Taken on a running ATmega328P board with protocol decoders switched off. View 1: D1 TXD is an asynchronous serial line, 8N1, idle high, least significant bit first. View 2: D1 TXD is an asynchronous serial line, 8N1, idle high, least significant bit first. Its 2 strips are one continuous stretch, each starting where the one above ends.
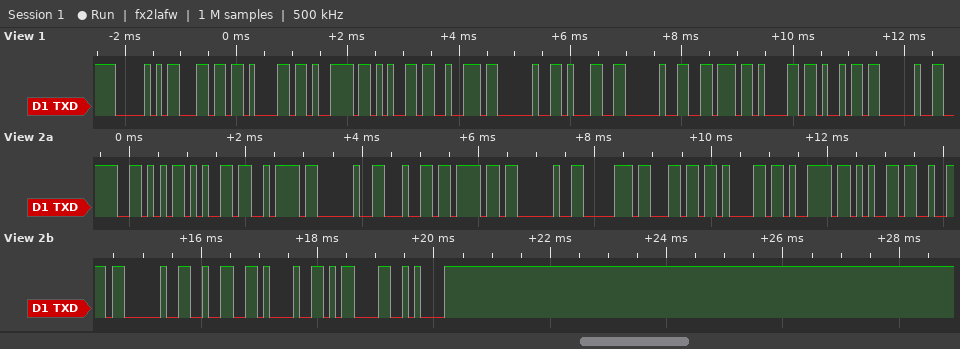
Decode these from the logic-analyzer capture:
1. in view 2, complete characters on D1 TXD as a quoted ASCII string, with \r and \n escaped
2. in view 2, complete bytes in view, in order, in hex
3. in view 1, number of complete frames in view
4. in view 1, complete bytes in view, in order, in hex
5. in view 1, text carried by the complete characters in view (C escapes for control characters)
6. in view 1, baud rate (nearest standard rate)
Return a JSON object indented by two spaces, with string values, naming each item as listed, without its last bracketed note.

{
  "in view 2, complete characters on D1 TXD as a quoted ASCII string, with \\r and \\n escaped": "\"Vez do player 2!\\r\\n\"",
  "in view 2, complete bytes in view, in order, in hex": "0x56 0x65 0x7A 0x20 0x64 0x6F 0x20 0x70 0x6C 0x61 0x79 0x65 0x72 0x20 0x32 0x21 0x0D 0x0A",
  "in view 1, number of complete frames in view": "13",
  "in view 1, complete bytes in view, in order, in hex": "50 6C 61 79 65 72 20 31 20 76 61 69 20",
  "in view 1, text carried by the complete characters in view": "\"Player 1 vai \"",
  "in view 1, baud rate": "9600 baud"
}
